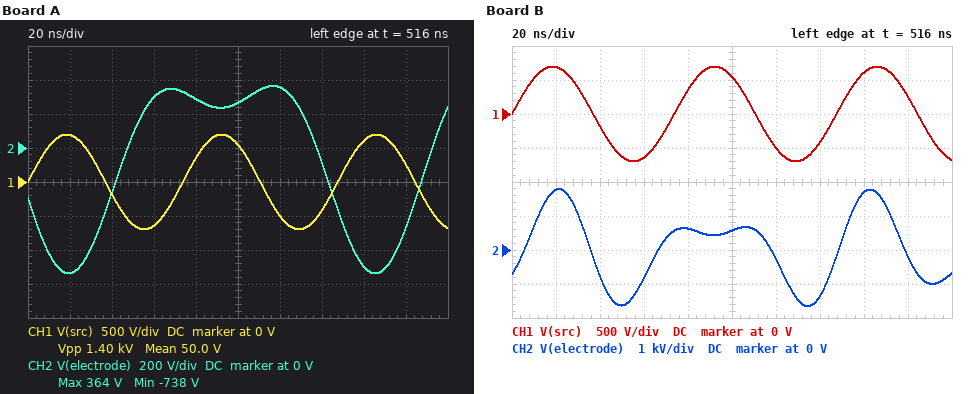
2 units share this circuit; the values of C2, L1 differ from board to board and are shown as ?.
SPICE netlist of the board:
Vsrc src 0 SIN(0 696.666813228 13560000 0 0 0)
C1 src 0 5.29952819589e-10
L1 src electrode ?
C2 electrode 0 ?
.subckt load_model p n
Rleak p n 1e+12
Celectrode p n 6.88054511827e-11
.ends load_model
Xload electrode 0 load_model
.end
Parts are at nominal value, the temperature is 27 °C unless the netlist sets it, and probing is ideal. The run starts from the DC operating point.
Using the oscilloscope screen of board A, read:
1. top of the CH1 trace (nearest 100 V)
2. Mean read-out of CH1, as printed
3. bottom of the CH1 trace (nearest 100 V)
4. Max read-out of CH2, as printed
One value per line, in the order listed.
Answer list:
700 V
50.0 V
-700 V
364 V
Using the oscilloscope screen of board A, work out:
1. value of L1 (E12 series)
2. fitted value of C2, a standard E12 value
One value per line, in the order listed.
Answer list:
1.8 µH
220 pF
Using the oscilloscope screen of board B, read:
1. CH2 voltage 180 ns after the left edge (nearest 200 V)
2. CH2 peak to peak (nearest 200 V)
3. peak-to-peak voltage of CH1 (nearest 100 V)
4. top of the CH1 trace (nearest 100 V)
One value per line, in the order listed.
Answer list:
-200 V
3.4 kV
1.4 kV
700 V
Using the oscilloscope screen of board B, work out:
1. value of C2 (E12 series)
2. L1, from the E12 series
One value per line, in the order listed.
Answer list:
68 pF
390 nH
